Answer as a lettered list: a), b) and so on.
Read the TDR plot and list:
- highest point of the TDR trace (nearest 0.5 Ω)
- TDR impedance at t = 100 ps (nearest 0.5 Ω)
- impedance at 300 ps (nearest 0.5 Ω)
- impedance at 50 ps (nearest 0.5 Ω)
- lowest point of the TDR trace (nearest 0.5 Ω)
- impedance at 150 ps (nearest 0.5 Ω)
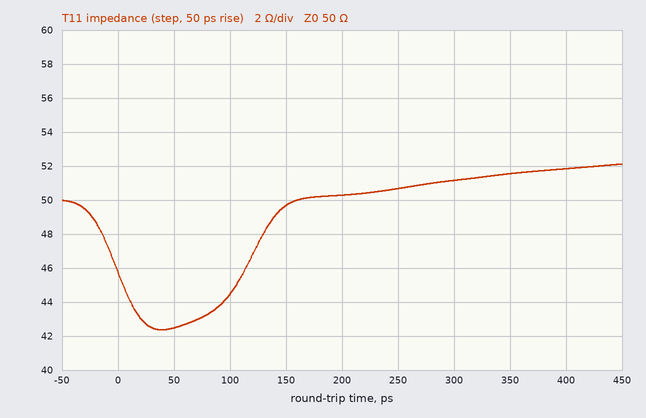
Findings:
a) 52.0 Ω
b) 44.5 Ω
c) 51.0 Ω
d) 42.5 Ω
e) 42.5 Ω
f) 49.5 Ω
